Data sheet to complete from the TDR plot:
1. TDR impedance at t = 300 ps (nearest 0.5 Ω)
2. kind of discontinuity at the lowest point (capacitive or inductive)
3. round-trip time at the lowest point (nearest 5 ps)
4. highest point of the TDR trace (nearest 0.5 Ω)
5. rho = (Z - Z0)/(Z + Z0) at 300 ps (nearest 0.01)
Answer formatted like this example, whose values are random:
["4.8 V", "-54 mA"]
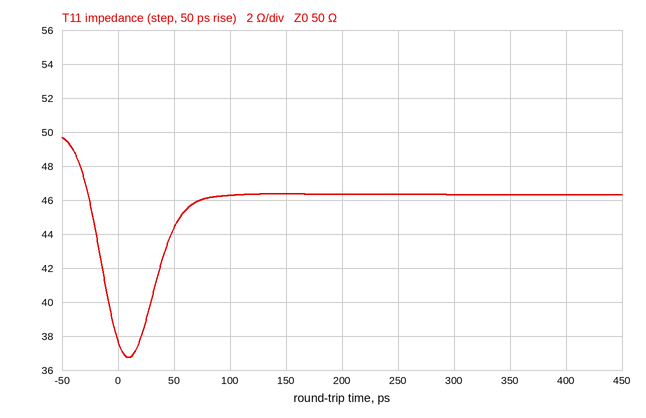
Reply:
["46.5 Ω", "capacitive", "10 ps", "49.5 Ω", "-0.04"]
